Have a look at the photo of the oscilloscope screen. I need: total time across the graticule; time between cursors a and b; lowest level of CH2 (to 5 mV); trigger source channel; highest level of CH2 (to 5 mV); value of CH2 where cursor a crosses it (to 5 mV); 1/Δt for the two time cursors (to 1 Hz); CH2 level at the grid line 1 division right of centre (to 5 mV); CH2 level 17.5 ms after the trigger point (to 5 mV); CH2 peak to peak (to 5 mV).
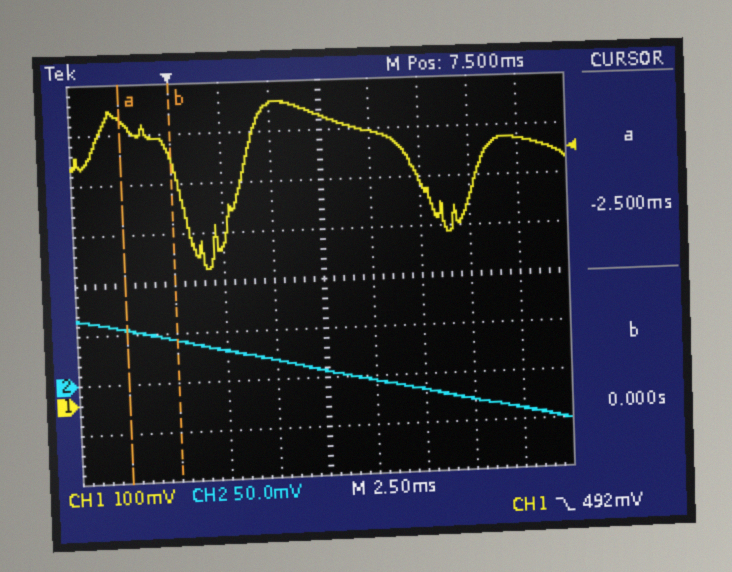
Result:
25 ms
2.50 ms
-50 mV
CH1
65 mV
55 mV
400 Hz
-5 mV
-40 mV
115 mV
